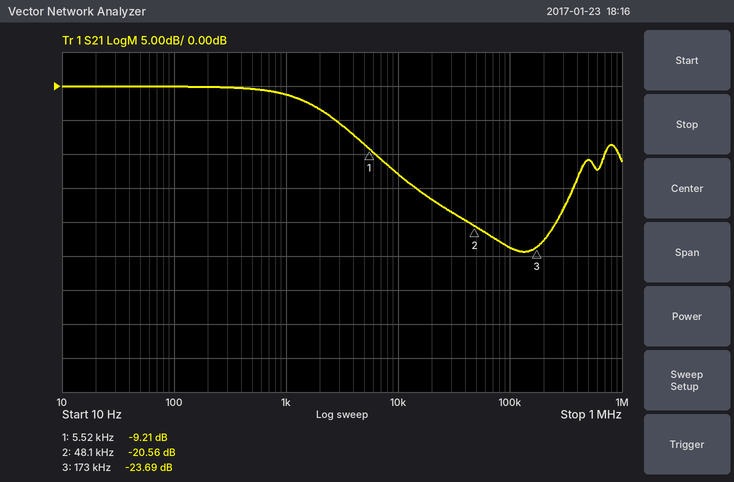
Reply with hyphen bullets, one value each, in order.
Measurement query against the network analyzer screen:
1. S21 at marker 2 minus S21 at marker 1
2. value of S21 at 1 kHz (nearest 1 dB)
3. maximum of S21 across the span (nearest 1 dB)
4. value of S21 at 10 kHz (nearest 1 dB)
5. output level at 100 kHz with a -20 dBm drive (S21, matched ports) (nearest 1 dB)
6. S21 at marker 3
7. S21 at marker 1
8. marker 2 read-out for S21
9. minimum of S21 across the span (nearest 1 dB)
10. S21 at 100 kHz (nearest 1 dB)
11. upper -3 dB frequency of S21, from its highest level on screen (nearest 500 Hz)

- -11.35 dB
- -1 dB
- 0 dB
- -13 dB
- -44 dBm
- -23.69 dB
- -9.21 dB
- -20.56 dB
- -24 dB
- -24 dB
- 2.0 kHz
